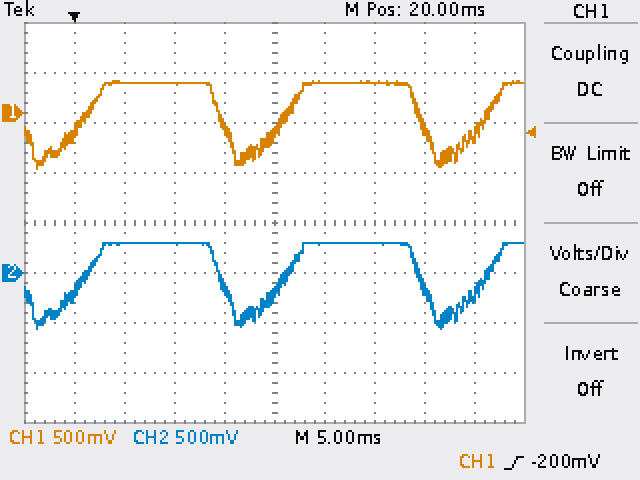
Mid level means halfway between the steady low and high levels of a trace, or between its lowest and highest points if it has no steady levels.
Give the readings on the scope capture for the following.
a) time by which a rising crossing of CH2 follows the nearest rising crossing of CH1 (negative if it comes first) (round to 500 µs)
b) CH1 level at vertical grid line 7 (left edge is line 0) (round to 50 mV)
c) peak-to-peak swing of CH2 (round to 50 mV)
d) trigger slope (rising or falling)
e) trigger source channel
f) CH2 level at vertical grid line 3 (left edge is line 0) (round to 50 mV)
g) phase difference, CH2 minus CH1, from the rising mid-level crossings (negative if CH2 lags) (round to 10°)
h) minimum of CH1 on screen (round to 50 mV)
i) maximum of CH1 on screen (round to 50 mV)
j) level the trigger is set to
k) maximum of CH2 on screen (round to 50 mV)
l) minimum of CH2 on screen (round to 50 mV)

0.0 ms
300 mV
850 mV
rising
CH1
300 mV
0°
-550 mV
300 mV
-200 mV
300 mV
-550 mV
